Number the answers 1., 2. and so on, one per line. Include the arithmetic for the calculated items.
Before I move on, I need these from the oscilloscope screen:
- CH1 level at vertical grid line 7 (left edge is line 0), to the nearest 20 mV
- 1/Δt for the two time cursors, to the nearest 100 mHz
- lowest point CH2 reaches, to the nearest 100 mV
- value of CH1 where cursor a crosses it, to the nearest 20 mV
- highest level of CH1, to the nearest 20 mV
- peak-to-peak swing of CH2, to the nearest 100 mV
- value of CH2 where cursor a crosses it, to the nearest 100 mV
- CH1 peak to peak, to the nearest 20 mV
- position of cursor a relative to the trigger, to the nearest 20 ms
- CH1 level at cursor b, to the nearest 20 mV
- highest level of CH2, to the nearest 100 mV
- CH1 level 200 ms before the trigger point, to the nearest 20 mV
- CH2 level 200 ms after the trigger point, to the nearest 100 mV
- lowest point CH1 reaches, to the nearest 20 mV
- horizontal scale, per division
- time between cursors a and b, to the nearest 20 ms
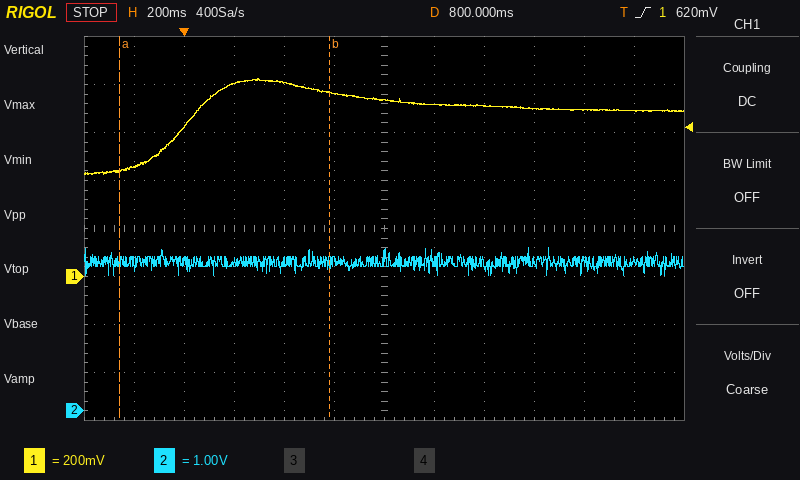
1. 720 mV
2. 1 / 840 ms ≈ 1.2 Hz
3. 2.8 V
4. 440 mV
5. 820 mV
6. 3.4 V − (2.8 V) = 600 mV
7. 3.1 V
8. 820 mV − (420 mV) = 400 mV
9. -260 ms
10. 760 mV
11. 3.4 V
12. 460 mV
13. 3.1 V
14. 420 mV
15. 200 ms
16. 840 ms
